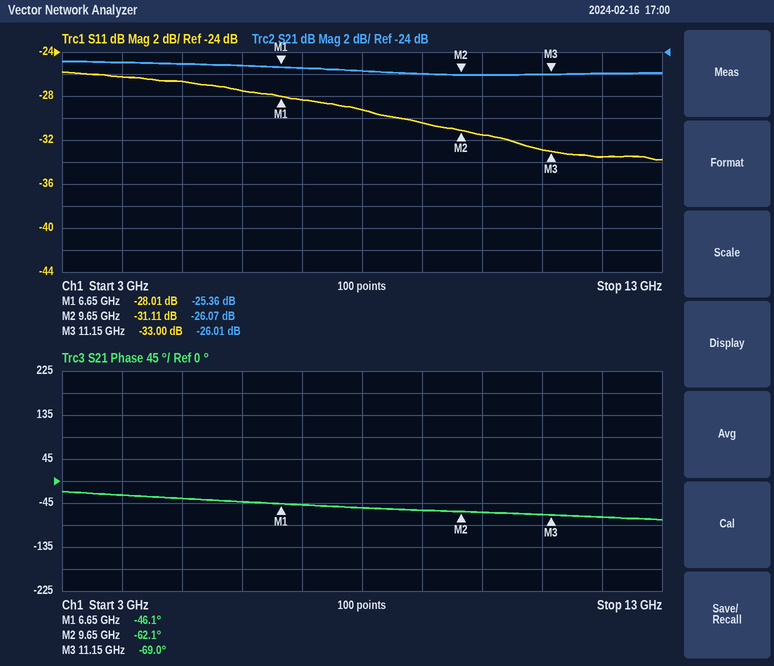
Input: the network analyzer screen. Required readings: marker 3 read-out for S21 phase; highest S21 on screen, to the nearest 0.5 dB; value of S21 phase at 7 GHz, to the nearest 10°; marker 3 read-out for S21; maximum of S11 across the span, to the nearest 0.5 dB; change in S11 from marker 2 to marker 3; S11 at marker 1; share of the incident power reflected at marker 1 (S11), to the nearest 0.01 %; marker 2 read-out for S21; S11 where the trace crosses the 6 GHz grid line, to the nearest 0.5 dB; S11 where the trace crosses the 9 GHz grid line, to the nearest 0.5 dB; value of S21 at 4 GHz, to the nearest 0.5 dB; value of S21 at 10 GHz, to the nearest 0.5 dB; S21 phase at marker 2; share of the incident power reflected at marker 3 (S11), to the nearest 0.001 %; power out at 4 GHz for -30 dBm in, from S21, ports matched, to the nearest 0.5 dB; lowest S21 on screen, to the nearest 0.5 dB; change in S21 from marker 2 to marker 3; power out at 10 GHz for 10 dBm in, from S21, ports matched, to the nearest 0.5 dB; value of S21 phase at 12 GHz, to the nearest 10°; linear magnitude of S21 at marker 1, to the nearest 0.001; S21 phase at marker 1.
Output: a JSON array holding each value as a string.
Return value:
["-69.0°", "-25.0 dB", "-50°", "-26.01 dB", "-26.0 dB", "-1.89 dB", "-28.01 dB", "0.16 %", "-26.07 dB", "-27.5 dB", "-30.5 dB", "-25.0 dB", "-26.0 dB", "-62.1°", "0.050 %", "-55.0 dBm", "-26.0 dB", "0.06 dB", "-16.0 dBm", "-70°", "0.054", "-46.1°"]
